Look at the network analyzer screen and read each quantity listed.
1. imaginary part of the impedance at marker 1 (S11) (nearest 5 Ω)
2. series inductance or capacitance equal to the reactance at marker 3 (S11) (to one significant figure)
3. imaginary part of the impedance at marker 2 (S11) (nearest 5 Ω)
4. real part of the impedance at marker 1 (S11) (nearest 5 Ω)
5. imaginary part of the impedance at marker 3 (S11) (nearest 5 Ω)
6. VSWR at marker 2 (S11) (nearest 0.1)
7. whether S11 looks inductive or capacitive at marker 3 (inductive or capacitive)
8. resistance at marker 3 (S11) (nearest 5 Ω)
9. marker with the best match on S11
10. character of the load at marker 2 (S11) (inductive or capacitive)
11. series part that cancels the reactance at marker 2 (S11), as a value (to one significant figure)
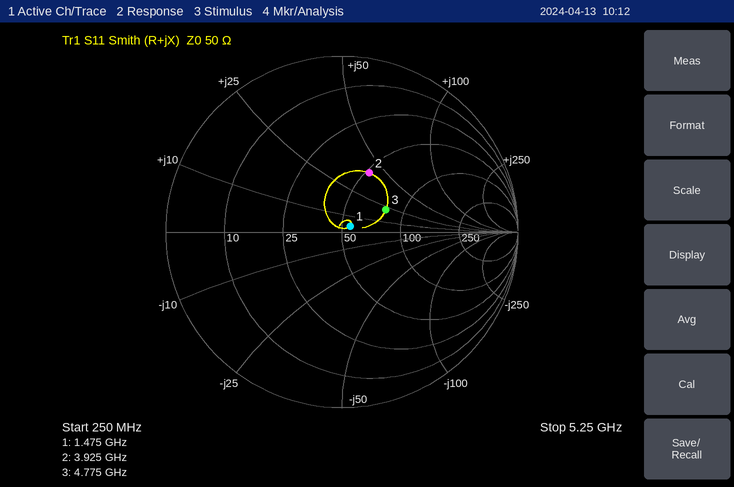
+5 Ω
700 pH
+40 Ω
55 Ω
+20 Ω
2.2
inductive
80 Ω
marker 1
inductive
1.0 pF
